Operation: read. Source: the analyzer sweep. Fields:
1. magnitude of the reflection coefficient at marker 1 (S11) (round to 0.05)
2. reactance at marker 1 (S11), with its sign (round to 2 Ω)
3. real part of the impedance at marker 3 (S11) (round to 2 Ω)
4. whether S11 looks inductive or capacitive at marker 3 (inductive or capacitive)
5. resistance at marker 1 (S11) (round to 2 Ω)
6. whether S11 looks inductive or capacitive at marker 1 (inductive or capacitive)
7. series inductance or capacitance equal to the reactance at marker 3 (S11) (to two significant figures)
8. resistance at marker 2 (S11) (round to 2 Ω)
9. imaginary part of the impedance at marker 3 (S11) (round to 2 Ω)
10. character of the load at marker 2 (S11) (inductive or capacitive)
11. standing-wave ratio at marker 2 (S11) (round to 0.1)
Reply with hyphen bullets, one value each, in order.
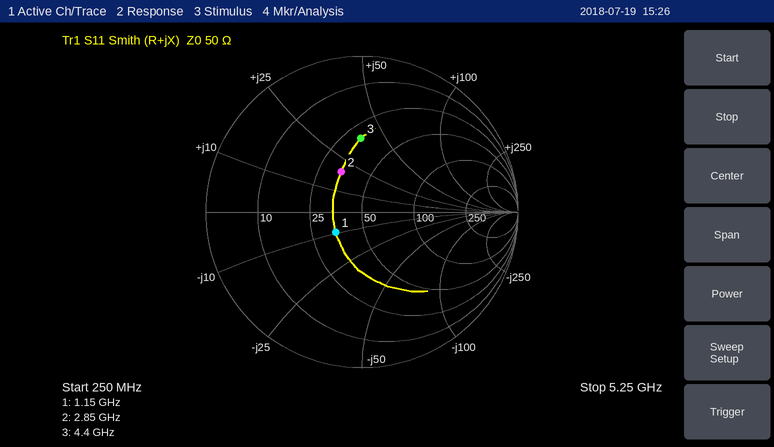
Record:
- 0.20
- -10 Ω
- 32 Ω
- inductive
- 34 Ω
- capacitive
- 1.4 nH
- 34 Ω
- +38 Ω
- inductive
- 1.8
